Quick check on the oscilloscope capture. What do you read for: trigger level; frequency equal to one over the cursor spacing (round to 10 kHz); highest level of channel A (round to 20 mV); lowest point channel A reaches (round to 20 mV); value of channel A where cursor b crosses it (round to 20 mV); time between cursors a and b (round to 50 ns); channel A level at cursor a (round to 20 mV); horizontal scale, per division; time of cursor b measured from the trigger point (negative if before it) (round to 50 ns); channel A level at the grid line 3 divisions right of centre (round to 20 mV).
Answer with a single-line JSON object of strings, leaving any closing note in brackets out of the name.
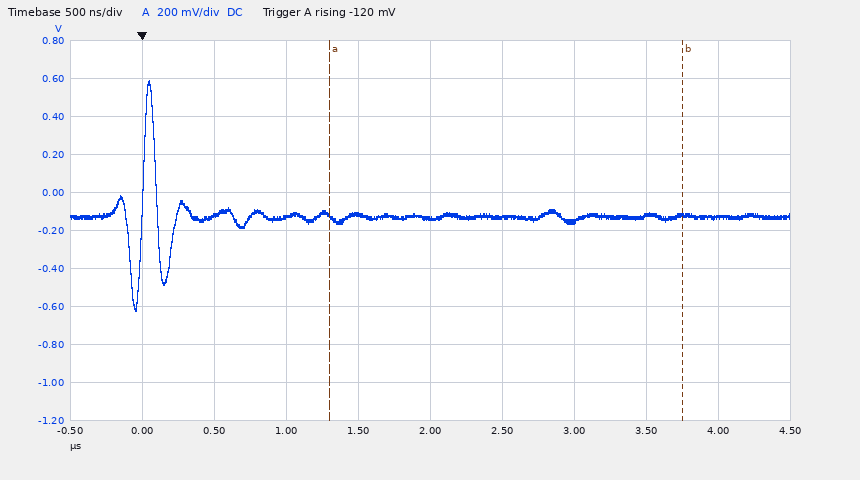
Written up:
{"trigger level": "-120 mV", "frequency equal to one over the cursor spacing": "410 kHz", "highest level of channel A": "580 mV", "lowest point channel A reaches": "-620 mV", "value of channel A where cursor b crosses it": "-120 mV", "time between cursors a and b": "2.45 µs", "channel A level at cursor a": "-120 mV", "horizontal scale, per division": "500 ns", "time of cursor b measured from the trigger point (negative if before it)": "+3.75 µs", "channel A level at the grid line 3 divisions right of centre": "-120 mV"}
